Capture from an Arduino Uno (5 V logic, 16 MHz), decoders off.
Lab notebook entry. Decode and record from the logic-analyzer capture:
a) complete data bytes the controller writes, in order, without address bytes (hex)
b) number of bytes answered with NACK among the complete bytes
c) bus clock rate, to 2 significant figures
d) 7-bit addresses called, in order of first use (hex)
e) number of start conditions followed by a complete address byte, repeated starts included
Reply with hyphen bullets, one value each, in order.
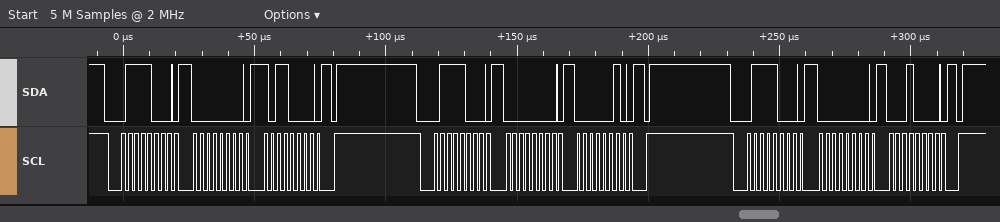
- 00 B0 00 02 00 10
- 0
- 400 kHz
- 0x3C
- 3
